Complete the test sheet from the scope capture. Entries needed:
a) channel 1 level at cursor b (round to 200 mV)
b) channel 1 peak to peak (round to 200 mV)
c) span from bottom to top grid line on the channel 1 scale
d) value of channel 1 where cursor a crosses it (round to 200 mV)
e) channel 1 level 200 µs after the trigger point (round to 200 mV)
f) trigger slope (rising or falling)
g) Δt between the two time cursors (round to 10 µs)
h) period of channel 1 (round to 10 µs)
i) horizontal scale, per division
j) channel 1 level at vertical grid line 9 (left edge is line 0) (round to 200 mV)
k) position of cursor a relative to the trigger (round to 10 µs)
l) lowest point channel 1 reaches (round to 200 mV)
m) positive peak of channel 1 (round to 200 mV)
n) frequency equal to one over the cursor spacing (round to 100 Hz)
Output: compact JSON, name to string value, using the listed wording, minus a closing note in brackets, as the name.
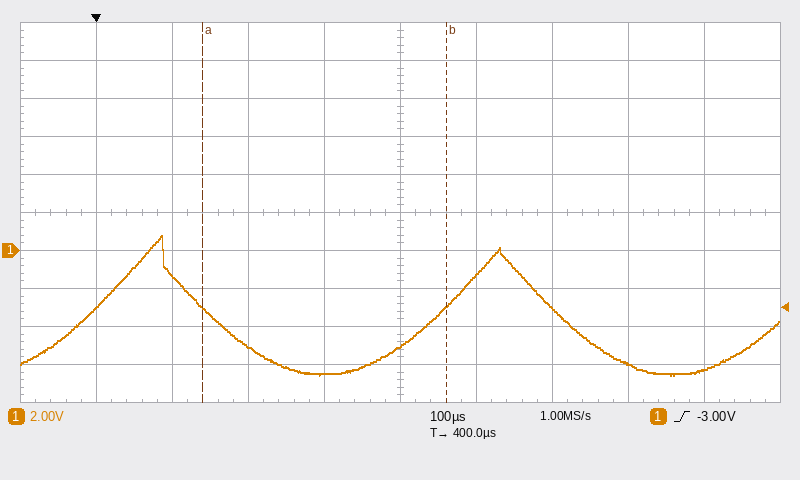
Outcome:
{"channel 1 level at cursor b": "-3.0 V", "channel 1 peak to peak": "7.4 V", "span from bottom to top grid line on the channel 1 scale": "20 V", "value of channel 1 where cursor a crosses it": "-3.0 V", "channel 1 level 200 µs after the trigger point": "-5.0 V", "trigger slope": "rising", "Δt between the two time cursors": "320 µs", "period of channel 1": "460 µs", "horizontal scale, per division": "100 µs", "channel 1 level at vertical grid line 9 (left edge is line 0)": "-6.2 V", "position of cursor a relative to the trigger": "+140 µs", "lowest point channel 1 reaches": "-6.6 V", "positive peak of channel 1": "800 mV", "frequency equal to one over the cursor spacing": "3.1 kHz"}
